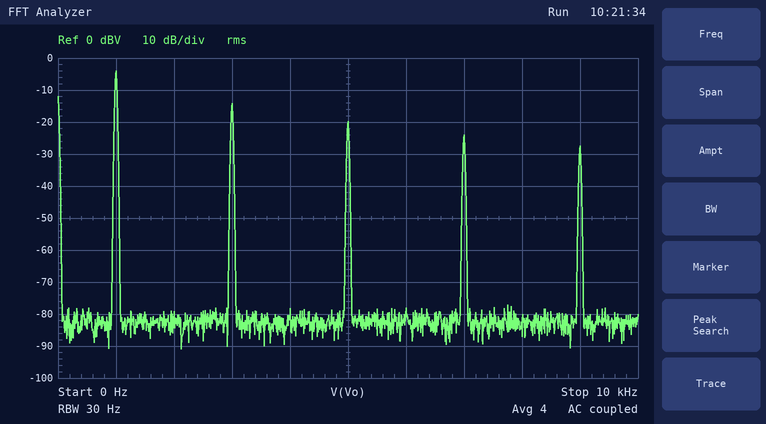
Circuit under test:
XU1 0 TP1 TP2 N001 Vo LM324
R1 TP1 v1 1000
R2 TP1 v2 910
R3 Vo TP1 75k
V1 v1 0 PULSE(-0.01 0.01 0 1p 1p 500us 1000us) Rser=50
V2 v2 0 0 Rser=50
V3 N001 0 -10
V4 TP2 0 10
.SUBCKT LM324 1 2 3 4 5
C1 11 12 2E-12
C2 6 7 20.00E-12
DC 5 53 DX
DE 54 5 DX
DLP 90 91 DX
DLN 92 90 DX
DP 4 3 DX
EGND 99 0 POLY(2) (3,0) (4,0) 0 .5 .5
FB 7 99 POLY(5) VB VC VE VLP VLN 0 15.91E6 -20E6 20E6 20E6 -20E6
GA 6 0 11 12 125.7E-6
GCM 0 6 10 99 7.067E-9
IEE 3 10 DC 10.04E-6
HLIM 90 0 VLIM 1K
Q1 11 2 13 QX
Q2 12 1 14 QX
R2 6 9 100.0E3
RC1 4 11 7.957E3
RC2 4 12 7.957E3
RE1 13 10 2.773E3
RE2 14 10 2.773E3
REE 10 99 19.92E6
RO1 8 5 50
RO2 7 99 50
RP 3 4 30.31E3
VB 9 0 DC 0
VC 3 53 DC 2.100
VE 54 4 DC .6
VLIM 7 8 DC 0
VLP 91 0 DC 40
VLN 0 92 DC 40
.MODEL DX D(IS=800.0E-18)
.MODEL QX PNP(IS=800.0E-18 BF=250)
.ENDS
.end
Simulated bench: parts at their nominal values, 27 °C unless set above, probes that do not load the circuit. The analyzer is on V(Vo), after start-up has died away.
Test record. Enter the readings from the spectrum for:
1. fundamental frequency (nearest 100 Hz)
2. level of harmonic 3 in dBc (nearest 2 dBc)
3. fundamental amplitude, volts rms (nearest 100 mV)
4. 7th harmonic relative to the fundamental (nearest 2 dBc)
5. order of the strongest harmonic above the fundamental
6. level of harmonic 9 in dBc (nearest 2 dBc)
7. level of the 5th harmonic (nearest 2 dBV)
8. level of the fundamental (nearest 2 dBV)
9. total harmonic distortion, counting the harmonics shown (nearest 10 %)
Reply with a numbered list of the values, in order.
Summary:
1. 1.0 kHz
2. -10 dBc
3. 600 mV
4. -20 dBc
5. 3
6. -24 dBc
7. -20 dBV
8. -4 dBV
9. 40 %
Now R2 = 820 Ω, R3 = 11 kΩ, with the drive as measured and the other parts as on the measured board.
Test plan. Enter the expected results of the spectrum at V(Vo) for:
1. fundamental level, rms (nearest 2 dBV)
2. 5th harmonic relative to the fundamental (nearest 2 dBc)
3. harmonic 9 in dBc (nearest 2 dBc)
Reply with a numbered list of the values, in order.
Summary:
1. -20 dBV
2. -14 dBc
3. -20 dBc
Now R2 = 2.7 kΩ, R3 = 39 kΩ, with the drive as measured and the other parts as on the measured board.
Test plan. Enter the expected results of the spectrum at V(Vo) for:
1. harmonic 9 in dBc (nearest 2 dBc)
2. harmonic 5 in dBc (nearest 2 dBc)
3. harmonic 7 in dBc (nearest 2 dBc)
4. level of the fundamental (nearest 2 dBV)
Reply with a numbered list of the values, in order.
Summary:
1. -20 dBc
2. -14 dBc
3. -18 dBc
4. -10 dBV
